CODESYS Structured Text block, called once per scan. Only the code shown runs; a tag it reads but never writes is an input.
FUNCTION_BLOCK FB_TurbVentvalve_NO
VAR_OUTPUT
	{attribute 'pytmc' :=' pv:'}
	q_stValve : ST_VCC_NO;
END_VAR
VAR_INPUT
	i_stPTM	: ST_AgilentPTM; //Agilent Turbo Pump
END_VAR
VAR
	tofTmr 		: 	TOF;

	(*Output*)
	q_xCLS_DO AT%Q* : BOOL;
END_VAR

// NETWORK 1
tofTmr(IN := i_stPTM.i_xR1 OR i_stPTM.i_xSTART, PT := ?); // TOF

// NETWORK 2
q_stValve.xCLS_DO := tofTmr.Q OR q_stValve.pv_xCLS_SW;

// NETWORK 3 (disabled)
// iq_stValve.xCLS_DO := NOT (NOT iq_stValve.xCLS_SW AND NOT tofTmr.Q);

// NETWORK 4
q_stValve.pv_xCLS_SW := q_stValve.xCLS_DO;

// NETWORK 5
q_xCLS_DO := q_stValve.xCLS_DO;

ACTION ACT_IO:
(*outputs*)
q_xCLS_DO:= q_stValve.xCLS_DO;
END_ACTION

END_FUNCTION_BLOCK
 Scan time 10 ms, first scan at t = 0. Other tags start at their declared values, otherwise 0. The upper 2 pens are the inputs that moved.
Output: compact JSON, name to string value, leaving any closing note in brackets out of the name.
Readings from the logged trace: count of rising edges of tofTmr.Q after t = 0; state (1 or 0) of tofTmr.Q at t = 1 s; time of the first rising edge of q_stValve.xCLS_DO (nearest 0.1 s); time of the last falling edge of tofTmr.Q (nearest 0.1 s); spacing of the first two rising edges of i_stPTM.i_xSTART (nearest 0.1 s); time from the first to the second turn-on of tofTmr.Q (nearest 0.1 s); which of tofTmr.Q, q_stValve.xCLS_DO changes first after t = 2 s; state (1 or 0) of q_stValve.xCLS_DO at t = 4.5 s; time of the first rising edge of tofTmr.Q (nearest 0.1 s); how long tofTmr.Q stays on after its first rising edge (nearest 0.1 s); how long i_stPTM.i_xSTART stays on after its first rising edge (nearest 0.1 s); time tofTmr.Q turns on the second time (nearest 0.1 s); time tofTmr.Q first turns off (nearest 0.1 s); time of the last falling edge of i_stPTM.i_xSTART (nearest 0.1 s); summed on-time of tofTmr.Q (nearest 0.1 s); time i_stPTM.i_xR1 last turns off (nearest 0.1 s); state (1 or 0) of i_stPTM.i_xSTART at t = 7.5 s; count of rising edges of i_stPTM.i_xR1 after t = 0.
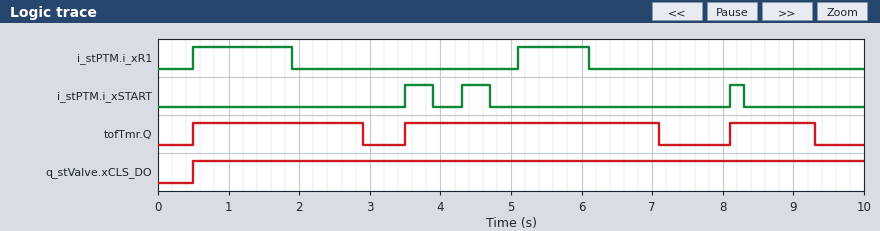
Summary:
{"count of rising edges of tofTmr.Q after t = 0": "3", "state (1 or 0) of tofTmr.Q at t = 1 s": "1", "time of the first rising edge of q_stValve.xCLS_DO": "0.5 s", "time of the last falling edge of tofTmr.Q": "9.3 s", "spacing of the first two rising edges of i_stPTM.i_xSTART": "0.8 s", "time from the first to the second turn-on of tofTmr.Q": "3.0 s", "which of tofTmr.Q, q_stValve.xCLS_DO changes first after t = 2 s": "tofTmr.Q", "state (1 or 0) of q_stValve.xCLS_DO at t = 4.5 s": "1", "time of the first rising edge of tofTmr.Q": "0.5 s", "how long tofTmr.Q stays on after its first rising edge": "2.4 s", "how long i_stPTM.i_xSTART stays on after its first rising edge": "0.4 s", "time tofTmr.Q turns on the second time": "3.5 s", "time tofTmr.Q first turns off": "2.9 s", "time of the last falling edge of i_stPTM.i_xSTART": "8.3 s", "summed on-time of tofTmr.Q": "7.2 s", "time i_stPTM.i_xR1 last turns off": "6.1 s", "state (1 or 0) of i_stPTM.i_xSTART at t = 7.5 s": "0", "count of rising edges of i_stPTM.i_xR1 after t = 0": "2"}
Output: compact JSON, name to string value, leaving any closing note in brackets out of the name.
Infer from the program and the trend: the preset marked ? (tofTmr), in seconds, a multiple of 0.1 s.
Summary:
{"the preset marked ? (tofTmr), in seconds, a multiple of 0.1 s": "1.0 s"}
